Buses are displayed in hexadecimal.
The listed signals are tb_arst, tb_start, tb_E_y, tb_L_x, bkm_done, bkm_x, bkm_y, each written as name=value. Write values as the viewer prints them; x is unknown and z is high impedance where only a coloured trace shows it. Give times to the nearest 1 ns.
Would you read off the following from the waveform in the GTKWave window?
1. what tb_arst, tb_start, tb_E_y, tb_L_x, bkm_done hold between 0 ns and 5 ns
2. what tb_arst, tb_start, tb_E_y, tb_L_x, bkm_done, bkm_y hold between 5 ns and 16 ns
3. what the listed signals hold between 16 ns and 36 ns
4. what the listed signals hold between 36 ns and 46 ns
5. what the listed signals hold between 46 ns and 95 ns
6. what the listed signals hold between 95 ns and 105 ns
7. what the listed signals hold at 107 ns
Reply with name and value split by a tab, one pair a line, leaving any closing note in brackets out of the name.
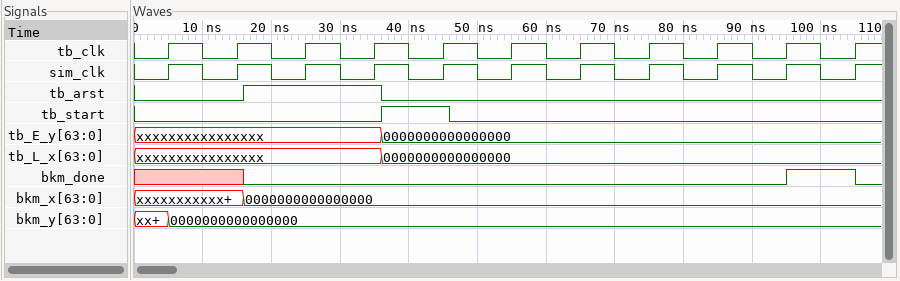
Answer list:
what tb_arst, tb_start, tb_E_y, tb_L_x, bkm_done hold between 0 ns and 5 ns	tb_arst=0, tb_start=0, tb_E_y=xxxxxxxxxxxxxxxx, tb_L_x=xxxxxxxxxxxxxxxx, bkm_done=x
what tb_arst, tb_start, tb_E_y, tb_L_x, bkm_done, bkm_y hold between 5 ns and 16 ns	tb_arst=0, tb_start=0, tb_E_y=xxxxxxxxxxxxxxxx, tb_L_x=xxxxxxxxxxxxxxxx, bkm_done=x, bkm_y=0000000000000000
what the listed signals hold between 16 ns and 36 ns	tb_arst=1, tb_start=0, tb_E_y=xxxxxxxxxxxxxxxx, tb_L_x=xxxxxxxxxxxxxxxx, bkm_done=0, bkm_x=0000000000000000, bkm_y=0000000000000000
what the listed signals hold between 36 ns and 46 ns	tb_arst=0, tb_start=1, tb_E_y=0000000000000000, tb_L_x=0000000000000000, bkm_done=0, bkm_x=0000000000000000, bkm_y=0000000000000000
what the listed signals hold between 46 ns and 95 ns	tb_arst=0, tb_start=0, tb_E_y=0000000000000000, tb_L_x=0000000000000000, bkm_done=0, bkm_x=0000000000000000, bkm_y=0000000000000000
what the listed signals hold between 95 ns and 105 ns	tb_arst=0, tb_start=0, tb_E_y=0000000000000000, tb_L_x=0000000000000000, bkm_done=1, bkm_x=0000000000000000, bkm_y=0000000000000000
what the listed signals hold at 107 ns	tb_arst=0, tb_start=0, tb_E_y=0000000000000000, tb_L_x=0000000000000000, bkm_done=0, bkm_x=0000000000000000, bkm_y=0000000000000000
